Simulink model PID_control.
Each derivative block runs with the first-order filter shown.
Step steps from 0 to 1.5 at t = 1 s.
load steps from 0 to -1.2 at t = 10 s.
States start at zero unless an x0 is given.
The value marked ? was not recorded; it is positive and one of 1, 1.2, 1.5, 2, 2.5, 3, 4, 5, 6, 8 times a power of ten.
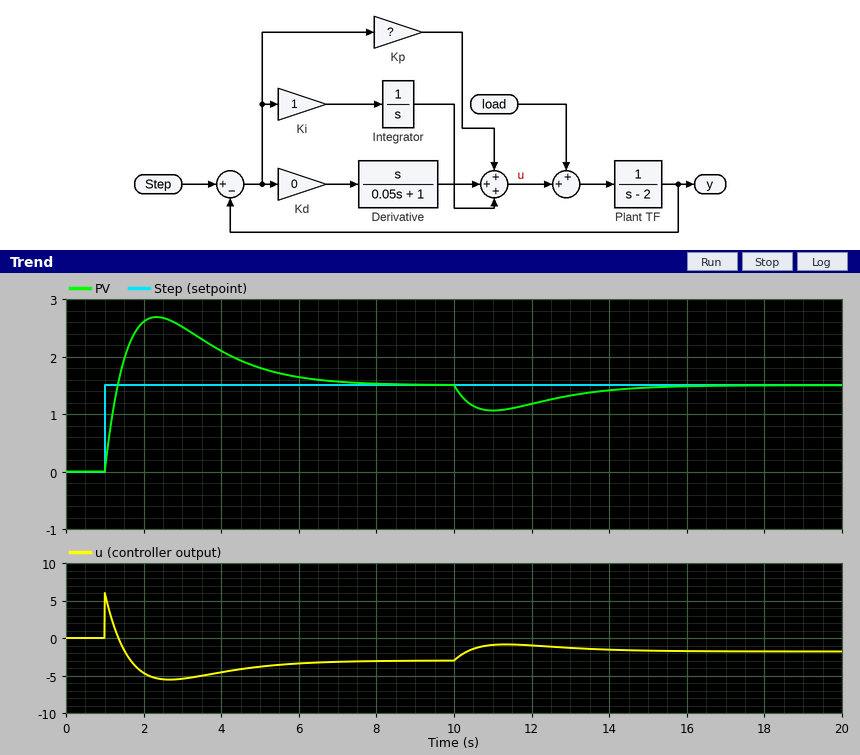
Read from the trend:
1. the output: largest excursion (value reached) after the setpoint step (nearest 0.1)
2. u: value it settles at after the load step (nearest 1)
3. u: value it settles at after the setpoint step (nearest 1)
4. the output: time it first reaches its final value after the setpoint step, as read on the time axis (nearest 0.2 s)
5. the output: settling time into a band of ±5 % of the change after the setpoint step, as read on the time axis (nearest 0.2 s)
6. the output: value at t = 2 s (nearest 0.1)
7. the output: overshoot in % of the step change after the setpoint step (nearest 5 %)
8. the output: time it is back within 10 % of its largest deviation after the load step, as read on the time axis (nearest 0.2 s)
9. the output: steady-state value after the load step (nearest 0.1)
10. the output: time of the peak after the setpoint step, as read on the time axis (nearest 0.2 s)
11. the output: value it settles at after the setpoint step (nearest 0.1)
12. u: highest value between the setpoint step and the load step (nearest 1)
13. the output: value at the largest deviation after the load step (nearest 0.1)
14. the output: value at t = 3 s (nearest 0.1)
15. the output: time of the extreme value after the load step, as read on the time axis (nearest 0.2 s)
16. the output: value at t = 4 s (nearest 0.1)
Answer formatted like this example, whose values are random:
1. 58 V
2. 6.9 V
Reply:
1. 2.7
2. -2
3. -3
4. 1.4 s
5. 6.8 s
6. 2.6
7. 80 %
8. 14.8 s
9. 1.5
10. 2.4 s
11. 1.5
12. 6
13. 1.1
14. 2.5
15. 11.0 s
16. 2.1
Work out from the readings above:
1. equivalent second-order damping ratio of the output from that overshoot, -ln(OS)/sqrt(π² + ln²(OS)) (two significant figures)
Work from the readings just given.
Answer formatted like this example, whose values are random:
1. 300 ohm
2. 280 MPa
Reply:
1. 0.071
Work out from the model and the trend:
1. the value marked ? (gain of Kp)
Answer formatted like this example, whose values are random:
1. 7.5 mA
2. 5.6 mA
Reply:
1. 4
